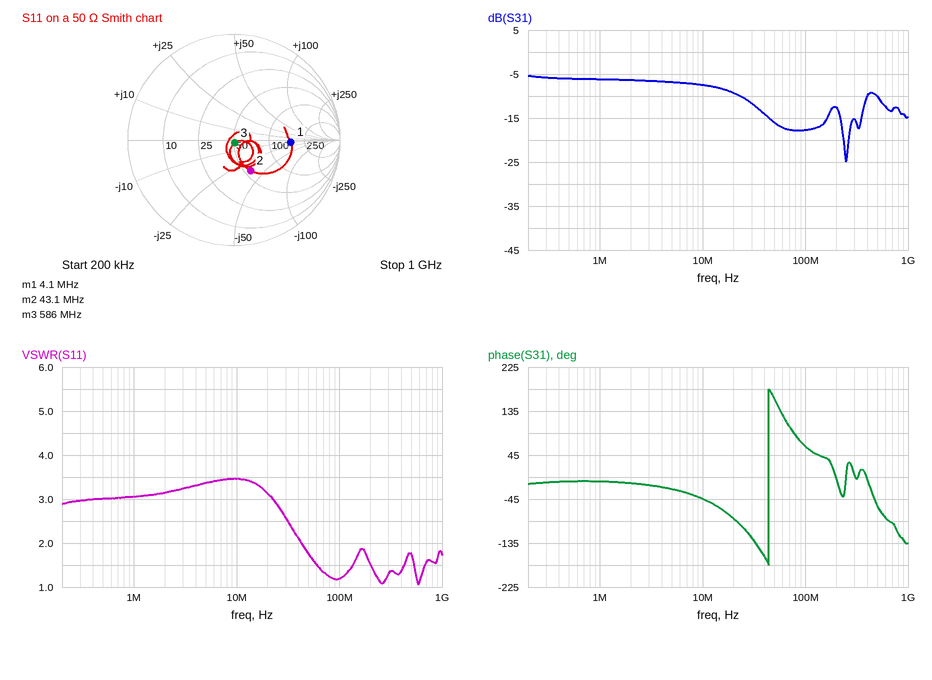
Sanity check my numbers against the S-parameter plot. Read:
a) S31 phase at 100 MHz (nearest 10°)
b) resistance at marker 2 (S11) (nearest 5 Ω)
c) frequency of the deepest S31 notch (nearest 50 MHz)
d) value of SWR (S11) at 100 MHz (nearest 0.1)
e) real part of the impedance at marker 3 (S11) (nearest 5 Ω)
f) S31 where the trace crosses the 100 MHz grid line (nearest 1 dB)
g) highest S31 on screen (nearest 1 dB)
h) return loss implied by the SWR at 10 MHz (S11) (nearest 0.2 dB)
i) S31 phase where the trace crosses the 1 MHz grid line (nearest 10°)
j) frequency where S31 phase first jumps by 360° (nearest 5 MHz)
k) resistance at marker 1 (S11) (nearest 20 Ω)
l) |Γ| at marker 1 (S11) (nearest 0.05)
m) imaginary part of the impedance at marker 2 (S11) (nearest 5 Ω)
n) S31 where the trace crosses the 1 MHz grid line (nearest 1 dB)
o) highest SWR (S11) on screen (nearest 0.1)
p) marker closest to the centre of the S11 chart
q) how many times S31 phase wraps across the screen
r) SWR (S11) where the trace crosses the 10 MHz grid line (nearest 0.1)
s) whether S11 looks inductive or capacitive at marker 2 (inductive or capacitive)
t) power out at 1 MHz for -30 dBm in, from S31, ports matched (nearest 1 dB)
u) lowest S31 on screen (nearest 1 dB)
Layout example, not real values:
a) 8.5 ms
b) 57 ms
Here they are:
a) 60°
b) 55 Ω
c) 250 MHz
d) 1.2
e) 50 Ω
f) -18 dB
g) -5 dB
h) 5.2 dB
i) -10°
j) 45 MHz
k) 160 Ω
l) 0.55
m) -35 Ω
n) -6 dB
o) 3.5
p) marker 3
q) 1
r) 3.5
s) capacitive
t) -36 dBm
u) -25 dB
